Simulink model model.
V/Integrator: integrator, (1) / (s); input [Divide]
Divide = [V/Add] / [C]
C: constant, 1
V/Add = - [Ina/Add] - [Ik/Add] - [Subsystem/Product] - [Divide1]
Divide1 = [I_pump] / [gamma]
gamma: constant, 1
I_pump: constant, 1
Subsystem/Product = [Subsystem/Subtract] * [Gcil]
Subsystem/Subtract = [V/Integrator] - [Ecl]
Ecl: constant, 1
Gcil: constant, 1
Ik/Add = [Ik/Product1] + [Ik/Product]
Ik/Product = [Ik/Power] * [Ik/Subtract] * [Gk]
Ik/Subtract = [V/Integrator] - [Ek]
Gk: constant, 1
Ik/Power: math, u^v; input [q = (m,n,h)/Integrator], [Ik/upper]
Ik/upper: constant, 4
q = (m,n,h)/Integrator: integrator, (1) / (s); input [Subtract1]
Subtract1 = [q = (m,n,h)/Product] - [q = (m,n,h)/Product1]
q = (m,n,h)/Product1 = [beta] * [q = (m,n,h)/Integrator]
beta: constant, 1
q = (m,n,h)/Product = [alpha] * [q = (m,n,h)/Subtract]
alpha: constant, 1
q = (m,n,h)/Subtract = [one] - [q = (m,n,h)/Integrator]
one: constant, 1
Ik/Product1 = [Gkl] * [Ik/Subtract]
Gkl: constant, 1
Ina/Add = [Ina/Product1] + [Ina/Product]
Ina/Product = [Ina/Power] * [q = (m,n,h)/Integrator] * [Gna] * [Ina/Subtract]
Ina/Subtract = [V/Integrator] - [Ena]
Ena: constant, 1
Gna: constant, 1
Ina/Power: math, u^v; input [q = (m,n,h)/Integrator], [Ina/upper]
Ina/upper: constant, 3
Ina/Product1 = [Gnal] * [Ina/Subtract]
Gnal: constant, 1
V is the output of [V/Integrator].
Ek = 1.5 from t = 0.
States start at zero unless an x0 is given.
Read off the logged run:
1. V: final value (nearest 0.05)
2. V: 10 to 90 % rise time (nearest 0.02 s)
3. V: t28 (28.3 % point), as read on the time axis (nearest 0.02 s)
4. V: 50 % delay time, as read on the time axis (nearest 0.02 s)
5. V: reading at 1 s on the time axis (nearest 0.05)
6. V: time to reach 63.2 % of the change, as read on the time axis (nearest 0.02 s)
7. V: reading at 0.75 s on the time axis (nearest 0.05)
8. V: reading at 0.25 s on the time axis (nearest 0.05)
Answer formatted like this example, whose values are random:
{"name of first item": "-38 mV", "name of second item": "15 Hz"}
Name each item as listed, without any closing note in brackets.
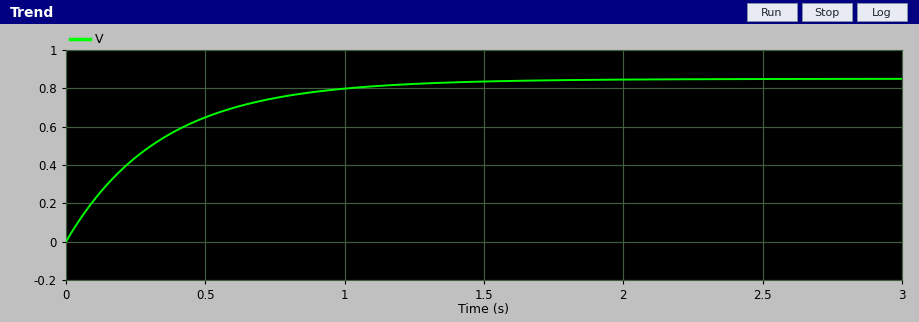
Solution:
{"V: final value": "0.85", "V: 10 to 90 % rise time": "0.78 s", "V: t28 (28.3 % point), as read on the time axis": "0.12 s", "V: 50 % delay time, as read on the time axis": "0.24 s", "V: reading at 1 s on the time axis": "0.80", "V: time to reach 63.2 % of the change, as read on the time axis": "0.34 s", "V: reading at 0.75 s on the time axis": "0.75", "V: reading at 0.25 s on the time axis": "0.45"}
